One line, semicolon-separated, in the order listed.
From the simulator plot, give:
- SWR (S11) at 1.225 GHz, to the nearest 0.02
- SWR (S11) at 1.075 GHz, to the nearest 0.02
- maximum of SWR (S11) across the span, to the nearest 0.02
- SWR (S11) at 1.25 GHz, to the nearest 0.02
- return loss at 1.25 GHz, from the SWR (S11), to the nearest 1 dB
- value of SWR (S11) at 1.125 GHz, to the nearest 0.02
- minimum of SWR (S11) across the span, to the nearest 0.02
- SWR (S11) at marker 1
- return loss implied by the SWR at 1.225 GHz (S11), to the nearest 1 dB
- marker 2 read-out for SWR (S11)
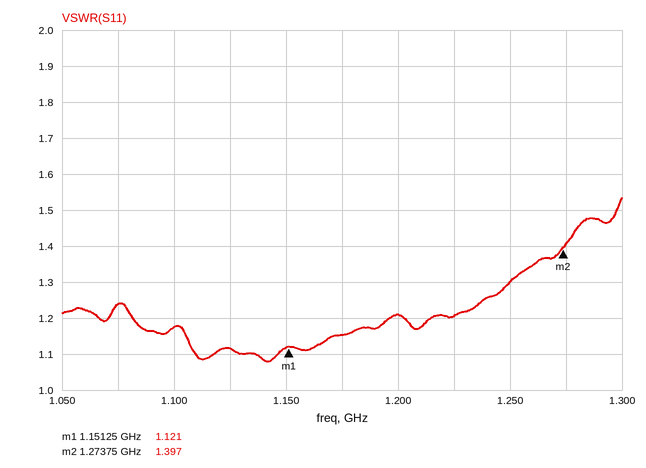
1.20; 1.24; 1.54; 1.30; 18 dB; 1.12; 1.08; 1.121; 21 dB; 1.397
